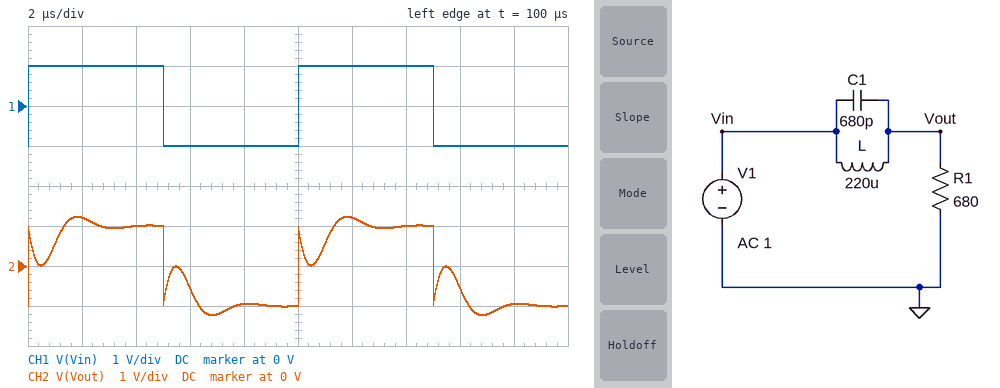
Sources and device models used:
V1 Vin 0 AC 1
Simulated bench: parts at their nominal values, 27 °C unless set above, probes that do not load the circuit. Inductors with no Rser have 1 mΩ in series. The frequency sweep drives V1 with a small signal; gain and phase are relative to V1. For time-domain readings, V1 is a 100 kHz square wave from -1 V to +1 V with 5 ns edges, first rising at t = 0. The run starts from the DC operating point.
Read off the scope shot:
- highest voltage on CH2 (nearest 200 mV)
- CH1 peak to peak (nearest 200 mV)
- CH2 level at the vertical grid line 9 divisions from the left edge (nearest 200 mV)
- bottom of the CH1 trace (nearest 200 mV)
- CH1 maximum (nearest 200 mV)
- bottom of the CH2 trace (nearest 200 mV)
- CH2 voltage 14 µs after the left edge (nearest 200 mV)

1.2 V
2.0 V
-1.0 V
-1.0 V
1.0 V
-1.2 V
1.0 V
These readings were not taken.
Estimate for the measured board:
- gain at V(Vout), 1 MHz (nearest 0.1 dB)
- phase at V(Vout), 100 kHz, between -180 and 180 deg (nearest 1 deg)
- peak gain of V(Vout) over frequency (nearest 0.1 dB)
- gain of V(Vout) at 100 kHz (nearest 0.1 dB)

-0.7 dB
-12 deg
0 dB
-0.2 dB
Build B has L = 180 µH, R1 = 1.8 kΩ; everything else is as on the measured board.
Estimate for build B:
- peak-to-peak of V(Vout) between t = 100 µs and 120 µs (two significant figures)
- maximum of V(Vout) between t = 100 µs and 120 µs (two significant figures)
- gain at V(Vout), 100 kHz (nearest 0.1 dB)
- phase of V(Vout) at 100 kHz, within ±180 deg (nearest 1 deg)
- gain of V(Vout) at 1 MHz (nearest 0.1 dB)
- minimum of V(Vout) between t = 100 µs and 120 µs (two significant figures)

2.6 V
1.3 V
0 dB
-4 deg
-0.1 dB
-1.3 V
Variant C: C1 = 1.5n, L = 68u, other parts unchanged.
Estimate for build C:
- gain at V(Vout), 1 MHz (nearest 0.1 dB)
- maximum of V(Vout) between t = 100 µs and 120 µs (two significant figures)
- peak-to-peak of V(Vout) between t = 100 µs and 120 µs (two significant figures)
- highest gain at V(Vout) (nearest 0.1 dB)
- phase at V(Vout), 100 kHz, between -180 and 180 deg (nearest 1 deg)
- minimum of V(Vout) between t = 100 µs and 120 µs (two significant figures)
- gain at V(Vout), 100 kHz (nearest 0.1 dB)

-0.2 dB
1.3 V
2.7 V
0 dB
-4 deg
-1.3 V
0 dB
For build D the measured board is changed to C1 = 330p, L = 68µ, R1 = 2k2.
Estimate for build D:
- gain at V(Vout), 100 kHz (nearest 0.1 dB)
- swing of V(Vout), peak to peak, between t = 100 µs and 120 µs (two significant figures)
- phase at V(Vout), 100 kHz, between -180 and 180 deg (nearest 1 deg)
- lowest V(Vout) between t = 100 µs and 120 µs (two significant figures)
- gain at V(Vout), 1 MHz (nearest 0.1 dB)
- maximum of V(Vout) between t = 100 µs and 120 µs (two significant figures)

0 dB
2.5 V
-1 deg
-1.3 V
-5.9 dB
1.3 V
